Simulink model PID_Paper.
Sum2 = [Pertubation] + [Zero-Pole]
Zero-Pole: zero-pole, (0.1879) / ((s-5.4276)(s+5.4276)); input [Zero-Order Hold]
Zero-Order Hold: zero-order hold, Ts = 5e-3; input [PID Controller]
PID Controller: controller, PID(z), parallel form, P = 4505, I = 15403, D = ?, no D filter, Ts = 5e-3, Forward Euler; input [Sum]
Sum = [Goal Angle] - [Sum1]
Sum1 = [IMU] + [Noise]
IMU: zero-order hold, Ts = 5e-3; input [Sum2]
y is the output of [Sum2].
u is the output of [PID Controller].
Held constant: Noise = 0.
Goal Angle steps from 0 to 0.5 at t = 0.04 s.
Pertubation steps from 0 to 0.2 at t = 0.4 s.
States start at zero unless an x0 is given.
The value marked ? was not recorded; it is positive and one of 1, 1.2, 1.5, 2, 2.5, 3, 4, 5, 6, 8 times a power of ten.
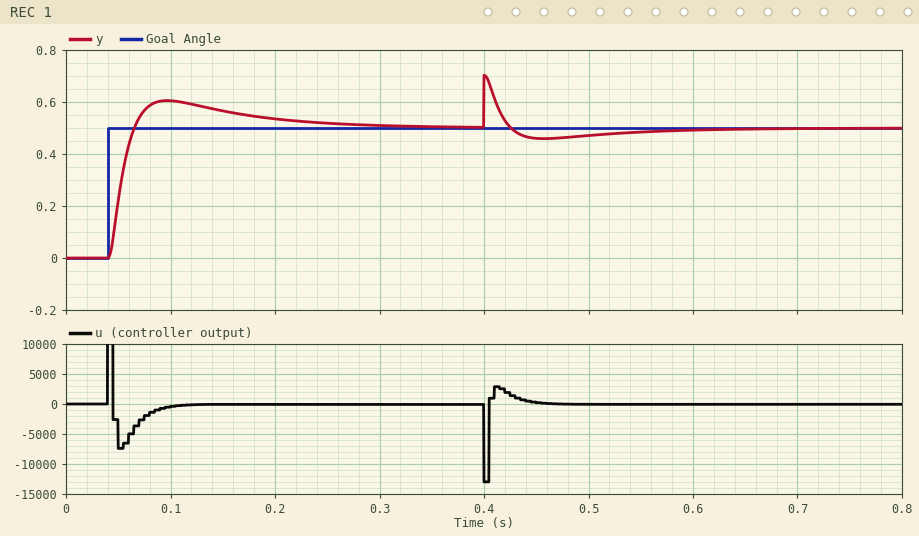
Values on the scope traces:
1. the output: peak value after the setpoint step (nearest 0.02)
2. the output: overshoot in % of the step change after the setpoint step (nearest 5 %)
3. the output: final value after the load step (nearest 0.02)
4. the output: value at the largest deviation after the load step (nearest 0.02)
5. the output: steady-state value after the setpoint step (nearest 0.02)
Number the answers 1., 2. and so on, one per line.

1. 0.60
2. 20 %
3. 0.50
4. 0.70
5. 0.50
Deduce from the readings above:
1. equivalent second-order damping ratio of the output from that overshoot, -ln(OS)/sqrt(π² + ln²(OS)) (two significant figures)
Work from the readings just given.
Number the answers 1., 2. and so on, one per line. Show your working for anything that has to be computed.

1. ln(0.2) = -1.609; 1.609 / sqrt(9.870 + 2.590) = 0.46
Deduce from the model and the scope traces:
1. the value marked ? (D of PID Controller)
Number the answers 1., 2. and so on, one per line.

1. 300
